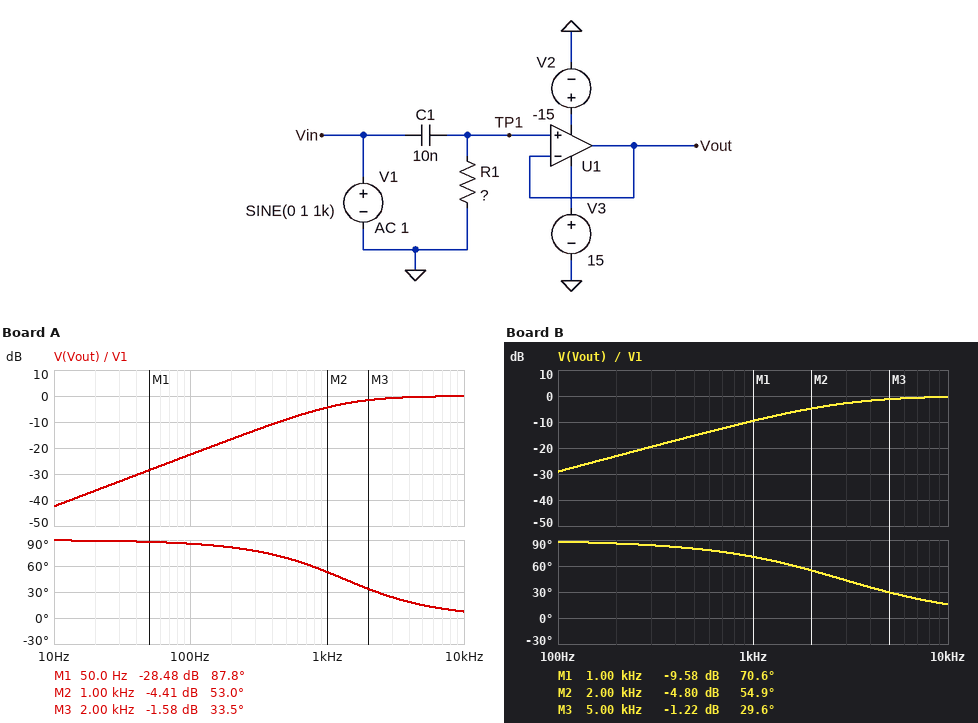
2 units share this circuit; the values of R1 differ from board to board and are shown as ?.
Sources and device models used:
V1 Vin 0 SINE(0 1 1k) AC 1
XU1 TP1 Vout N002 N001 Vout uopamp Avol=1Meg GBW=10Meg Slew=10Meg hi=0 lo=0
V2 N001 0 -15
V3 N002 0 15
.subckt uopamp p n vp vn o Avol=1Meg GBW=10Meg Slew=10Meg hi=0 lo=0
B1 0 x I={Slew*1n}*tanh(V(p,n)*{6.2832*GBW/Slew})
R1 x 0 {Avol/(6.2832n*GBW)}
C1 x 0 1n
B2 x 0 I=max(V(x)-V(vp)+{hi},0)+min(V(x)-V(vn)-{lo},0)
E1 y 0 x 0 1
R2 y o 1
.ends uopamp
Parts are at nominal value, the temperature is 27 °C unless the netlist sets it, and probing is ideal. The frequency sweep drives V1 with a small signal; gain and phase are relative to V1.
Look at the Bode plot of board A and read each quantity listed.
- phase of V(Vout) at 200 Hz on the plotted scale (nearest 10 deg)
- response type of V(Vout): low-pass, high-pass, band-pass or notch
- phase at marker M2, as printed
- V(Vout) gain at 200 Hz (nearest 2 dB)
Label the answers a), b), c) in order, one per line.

a) 80 deg
b) high-pass
c) 53.0 deg
d) -16 dB
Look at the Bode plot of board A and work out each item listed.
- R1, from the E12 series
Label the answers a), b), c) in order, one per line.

a) 12 kΩ
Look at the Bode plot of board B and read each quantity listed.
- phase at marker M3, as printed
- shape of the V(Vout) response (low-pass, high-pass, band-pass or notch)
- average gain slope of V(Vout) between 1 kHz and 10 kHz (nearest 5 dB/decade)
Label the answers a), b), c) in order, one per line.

a) 29.6 deg
b) high-pass
c) 10 dB/decade
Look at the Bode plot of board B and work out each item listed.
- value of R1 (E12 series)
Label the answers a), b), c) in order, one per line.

a) 5.6 kΩ
